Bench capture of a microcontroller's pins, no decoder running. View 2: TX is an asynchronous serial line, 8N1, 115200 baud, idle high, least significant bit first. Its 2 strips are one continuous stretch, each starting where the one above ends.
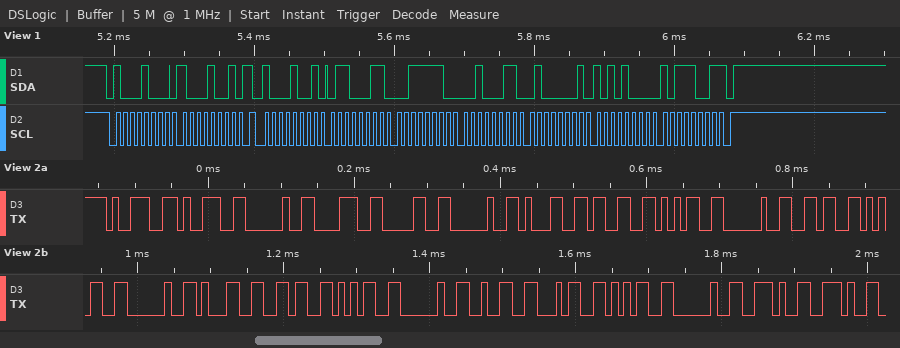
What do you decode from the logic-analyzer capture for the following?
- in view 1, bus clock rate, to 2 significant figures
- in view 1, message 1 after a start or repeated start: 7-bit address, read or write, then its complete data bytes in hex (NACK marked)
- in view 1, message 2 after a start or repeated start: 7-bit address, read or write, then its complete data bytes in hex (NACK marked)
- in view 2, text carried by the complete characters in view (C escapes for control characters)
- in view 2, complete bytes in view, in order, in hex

100 kHz
0x44 write: 89
0x44 read: 63 3E 23 41 A8 B9 NACK
"99 80 135 65 165 245 .."
0x39 0x39 0x20 0x38 0x30 0x20 0x31 0x33 0x35 0x20 0x36 0x35 0x20 0x31 0x36 0x35 0x20 0x32 0x34 0x35 0x20 0x2E 0x2E
